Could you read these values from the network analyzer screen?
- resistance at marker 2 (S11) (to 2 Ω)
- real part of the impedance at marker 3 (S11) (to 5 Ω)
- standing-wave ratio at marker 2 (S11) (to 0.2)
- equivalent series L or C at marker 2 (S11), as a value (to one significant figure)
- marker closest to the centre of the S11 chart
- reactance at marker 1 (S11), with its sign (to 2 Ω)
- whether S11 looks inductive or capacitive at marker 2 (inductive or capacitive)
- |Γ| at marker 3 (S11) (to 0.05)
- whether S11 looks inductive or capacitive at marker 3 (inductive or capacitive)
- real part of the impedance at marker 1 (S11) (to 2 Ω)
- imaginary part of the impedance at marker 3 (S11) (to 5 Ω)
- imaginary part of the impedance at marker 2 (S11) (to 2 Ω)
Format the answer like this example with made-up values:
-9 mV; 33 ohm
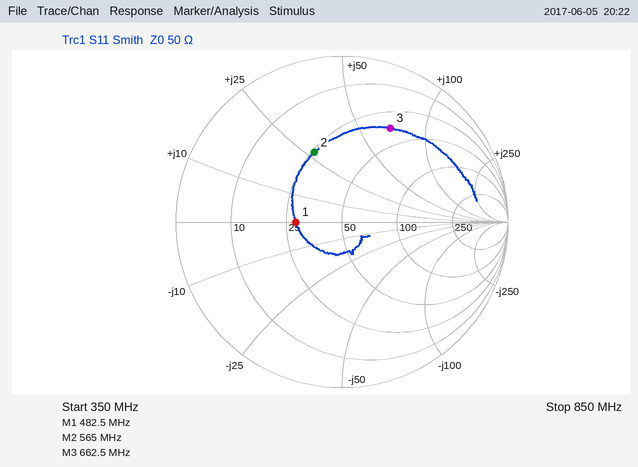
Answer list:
26 Ω; 35 Ω; 2.6; 8 nH; marker 1; 0 Ω; inductive; 0.65; inductive; 28 Ω; +70 Ω; +28 Ω
